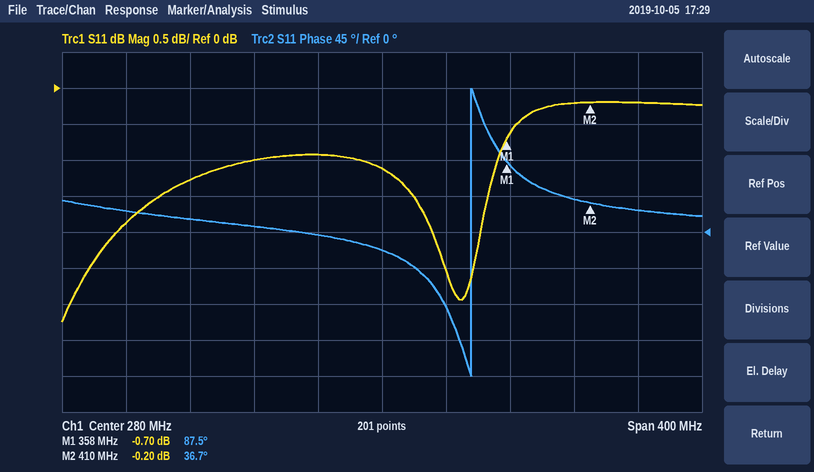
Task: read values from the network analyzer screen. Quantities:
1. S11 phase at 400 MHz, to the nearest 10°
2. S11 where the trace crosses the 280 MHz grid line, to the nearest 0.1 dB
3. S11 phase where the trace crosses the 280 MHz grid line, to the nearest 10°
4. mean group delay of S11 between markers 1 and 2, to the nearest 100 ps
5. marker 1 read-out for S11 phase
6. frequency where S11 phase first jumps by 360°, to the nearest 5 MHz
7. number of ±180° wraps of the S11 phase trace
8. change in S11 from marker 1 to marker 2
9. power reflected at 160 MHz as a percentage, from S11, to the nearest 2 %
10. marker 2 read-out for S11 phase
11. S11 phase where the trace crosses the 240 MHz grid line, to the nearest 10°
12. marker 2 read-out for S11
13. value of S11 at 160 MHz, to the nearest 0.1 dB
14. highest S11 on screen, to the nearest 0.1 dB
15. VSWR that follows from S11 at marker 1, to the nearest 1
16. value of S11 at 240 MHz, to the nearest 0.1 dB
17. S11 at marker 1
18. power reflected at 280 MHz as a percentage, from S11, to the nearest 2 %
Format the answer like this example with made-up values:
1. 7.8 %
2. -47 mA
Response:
1. 40°
2. -1.1 dB
3. -20°
4. 2.7 ns
5. 87.5°
6. 335 MHz
7. 1
8. 0.50 dB
9. 74 %
10. 36.7°
11. 0°
12. -0.20 dB
13. -1.3 dB
14. -0.2 dB
15. 25
16. -0.9 dB
17. -0.70 dB
18. 78 %
